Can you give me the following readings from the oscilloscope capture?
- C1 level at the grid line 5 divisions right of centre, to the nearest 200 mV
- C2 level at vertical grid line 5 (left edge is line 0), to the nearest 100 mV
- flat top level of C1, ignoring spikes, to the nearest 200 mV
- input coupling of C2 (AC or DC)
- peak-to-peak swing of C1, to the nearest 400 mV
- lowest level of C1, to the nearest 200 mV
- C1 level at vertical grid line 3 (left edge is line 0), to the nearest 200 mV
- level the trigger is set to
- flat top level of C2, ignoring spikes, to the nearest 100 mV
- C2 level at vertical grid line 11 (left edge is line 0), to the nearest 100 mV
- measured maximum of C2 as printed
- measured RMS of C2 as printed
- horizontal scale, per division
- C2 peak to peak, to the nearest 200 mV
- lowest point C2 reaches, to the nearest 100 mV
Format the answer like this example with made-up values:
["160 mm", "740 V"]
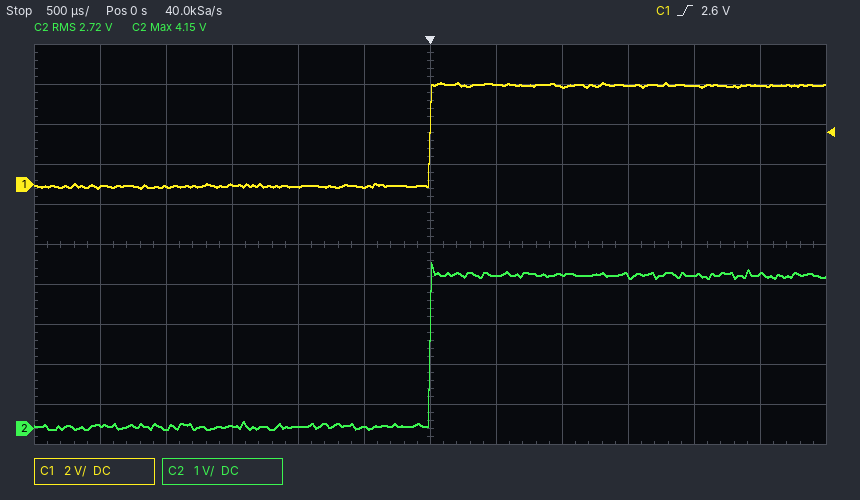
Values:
["5.0 V", "0.0 V", "5.0 V", "DC", "5.2 V", "-200 mV", "0.0 V", "2.6 V", "3.8 V", "3.9 V", "4.15 V", "2.72 V", "500 µs", "4.2 V", "0.0 V"]
